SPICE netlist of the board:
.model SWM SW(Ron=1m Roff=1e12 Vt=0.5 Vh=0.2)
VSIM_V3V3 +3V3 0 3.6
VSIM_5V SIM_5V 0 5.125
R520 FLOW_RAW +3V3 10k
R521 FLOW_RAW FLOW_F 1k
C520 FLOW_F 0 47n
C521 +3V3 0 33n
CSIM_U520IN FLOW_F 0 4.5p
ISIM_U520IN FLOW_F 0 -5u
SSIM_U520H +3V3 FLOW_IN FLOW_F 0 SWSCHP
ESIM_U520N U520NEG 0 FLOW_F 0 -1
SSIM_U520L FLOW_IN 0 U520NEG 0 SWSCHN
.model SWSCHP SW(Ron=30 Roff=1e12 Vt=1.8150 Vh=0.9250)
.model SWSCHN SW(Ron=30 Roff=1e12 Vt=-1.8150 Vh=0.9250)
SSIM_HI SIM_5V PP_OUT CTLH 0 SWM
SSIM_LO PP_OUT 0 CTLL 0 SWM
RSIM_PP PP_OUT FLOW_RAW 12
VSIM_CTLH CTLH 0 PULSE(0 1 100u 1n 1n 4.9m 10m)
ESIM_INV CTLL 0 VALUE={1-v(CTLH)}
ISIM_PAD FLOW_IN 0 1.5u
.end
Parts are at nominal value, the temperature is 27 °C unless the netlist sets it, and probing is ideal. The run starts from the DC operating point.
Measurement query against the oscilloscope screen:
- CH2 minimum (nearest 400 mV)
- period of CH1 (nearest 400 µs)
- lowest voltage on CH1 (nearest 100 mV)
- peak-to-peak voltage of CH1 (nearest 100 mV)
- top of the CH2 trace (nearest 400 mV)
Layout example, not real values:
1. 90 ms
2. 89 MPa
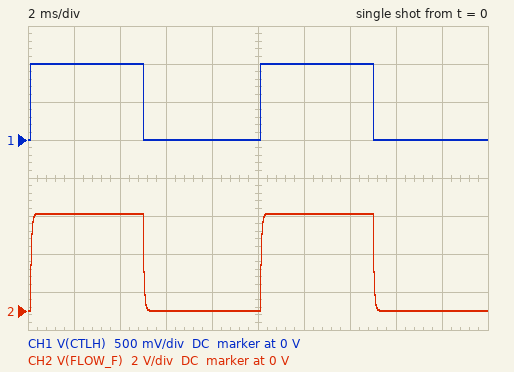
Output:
1. 0 V
2. 10.0 ms
3. 0 V
4. 1.0 V
5. 5.2 V
